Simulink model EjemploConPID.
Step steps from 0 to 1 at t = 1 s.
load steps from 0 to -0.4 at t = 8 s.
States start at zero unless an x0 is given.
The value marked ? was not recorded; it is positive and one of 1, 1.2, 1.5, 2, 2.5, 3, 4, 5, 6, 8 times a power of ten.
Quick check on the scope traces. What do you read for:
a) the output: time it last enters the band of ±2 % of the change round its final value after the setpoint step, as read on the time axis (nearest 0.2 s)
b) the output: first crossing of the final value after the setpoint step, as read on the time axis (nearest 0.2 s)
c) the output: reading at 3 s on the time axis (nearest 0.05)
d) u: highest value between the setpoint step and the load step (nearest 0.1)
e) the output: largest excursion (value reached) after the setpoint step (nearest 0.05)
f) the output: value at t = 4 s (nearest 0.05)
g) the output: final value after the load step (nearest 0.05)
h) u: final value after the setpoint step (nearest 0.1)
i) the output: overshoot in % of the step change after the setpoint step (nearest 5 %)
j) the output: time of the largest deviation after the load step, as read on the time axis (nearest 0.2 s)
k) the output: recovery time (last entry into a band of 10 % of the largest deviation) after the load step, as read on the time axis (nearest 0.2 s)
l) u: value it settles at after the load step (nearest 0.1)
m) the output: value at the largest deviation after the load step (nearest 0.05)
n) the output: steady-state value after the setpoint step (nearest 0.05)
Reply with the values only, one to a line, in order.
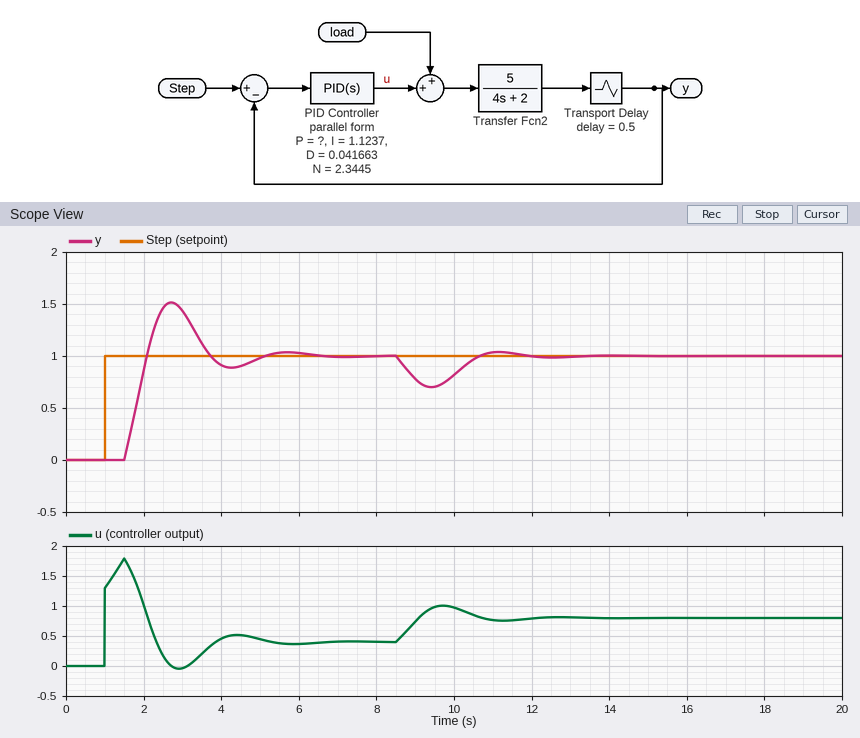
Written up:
6.2 s
2.0 s
1.45
1.8
1.50
0.90
1.00
0.4
50 %
9.4 s
11.4 s
0.8
0.70
1.00
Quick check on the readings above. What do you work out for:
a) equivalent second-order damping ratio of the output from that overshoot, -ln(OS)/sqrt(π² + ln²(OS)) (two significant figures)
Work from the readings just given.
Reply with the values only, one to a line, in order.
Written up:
0.22
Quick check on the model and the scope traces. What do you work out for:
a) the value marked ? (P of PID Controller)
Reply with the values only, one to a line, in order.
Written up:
1.2
